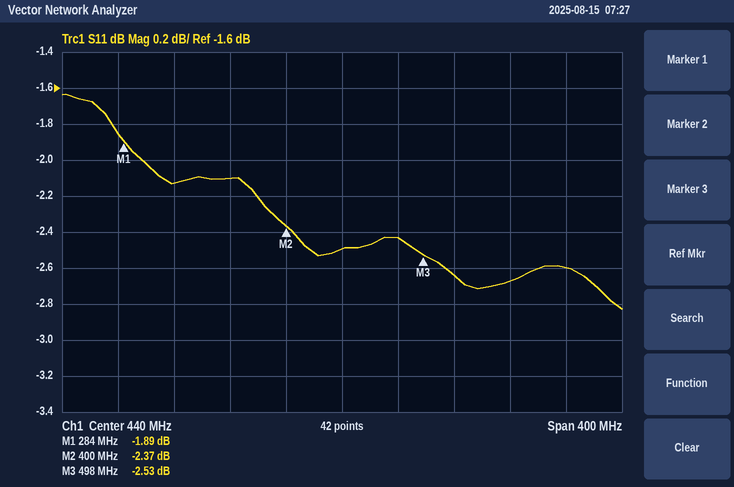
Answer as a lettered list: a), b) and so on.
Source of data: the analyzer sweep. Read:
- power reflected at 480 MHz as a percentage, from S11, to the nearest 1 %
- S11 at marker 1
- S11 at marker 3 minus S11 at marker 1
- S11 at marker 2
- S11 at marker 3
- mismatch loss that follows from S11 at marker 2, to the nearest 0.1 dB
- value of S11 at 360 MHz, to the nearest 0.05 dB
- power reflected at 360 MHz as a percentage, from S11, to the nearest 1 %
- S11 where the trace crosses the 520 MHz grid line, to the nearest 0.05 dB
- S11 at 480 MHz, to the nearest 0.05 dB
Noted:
a) 57 %
b) -1.89 dB
c) -0.64 dB
d) -2.37 dB
e) -2.53 dB
f) 3.8 dB
g) -2.10 dB
h) 62 %
i) -2.65 dB
j) -2.45 dB
